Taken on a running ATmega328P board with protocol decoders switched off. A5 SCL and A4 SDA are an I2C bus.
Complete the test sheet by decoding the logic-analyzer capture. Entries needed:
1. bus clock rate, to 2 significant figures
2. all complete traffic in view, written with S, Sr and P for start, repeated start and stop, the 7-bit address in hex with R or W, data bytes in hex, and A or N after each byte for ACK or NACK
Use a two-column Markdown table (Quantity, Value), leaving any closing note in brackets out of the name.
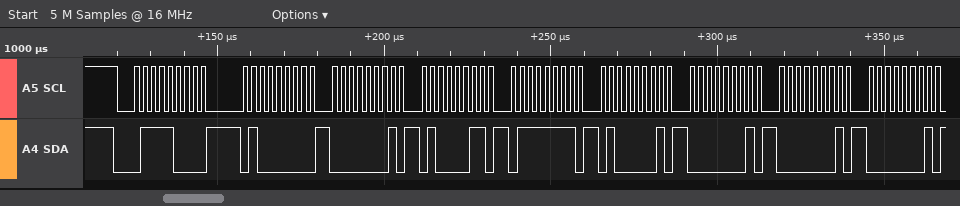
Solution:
| Quantity | Value |
|---|---|
| bus clock rate, to 2 significant figures | 400 kHz |
| all complete traffic in view, written with S, Sr and P for start, repeated start and stop, the 7-bit address in hex with R or W, data bytes in hex, and A or N after each byte for ACK or NACK | S 3CW A 40 A 01 A 43 A 7F A 41 A 01 A 01 A 01 A |
